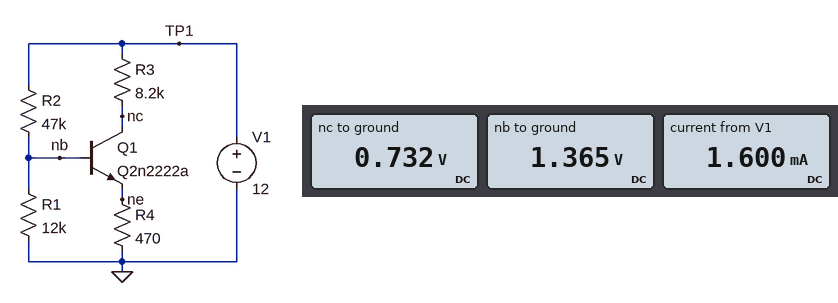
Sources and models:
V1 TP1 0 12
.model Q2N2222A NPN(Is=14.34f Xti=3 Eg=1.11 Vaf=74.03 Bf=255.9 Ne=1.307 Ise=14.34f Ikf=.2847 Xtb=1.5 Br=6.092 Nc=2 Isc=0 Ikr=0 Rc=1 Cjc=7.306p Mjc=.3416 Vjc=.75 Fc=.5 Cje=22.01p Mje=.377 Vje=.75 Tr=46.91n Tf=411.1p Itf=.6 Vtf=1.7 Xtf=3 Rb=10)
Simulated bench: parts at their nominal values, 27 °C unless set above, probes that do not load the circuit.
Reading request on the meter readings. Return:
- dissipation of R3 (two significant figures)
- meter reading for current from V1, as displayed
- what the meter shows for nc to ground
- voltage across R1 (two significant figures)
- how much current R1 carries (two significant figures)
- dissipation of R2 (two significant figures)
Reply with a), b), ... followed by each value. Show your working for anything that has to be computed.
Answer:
a) (12 V - 732 mV)^2 / 8.2 kΩ = 15 mW
b) 1.600 mA
c) 0.732 V
d) 1.365 V = 1.4 V
e) (1.365 V) / 12 kΩ = 110 µA
f) (12 V - 1.365 V)^2 / 47 kΩ = 2.4 mW
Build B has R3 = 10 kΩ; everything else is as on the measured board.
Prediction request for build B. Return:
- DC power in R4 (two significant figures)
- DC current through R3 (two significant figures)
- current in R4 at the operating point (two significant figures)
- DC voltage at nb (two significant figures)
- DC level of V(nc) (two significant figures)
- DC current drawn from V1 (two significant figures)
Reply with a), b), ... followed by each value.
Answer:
a) 750 µW
b) 1.1 mA
c) 1.3 mA
d) 1.3 V
e) 620 mV
f) 1.4 mA
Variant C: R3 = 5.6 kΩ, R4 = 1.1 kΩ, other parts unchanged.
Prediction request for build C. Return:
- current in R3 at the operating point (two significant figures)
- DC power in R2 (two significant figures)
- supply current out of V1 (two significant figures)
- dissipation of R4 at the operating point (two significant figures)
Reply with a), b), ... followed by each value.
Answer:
a) 1.5 mA
b) 2.0 mW
c) 1.7 mA
d) 2.6 mW
